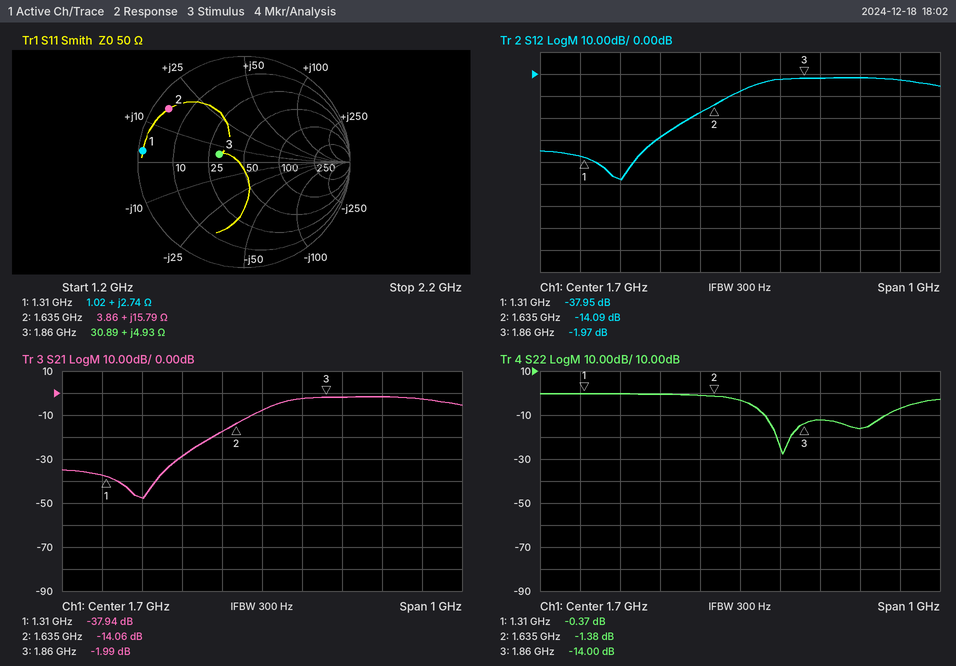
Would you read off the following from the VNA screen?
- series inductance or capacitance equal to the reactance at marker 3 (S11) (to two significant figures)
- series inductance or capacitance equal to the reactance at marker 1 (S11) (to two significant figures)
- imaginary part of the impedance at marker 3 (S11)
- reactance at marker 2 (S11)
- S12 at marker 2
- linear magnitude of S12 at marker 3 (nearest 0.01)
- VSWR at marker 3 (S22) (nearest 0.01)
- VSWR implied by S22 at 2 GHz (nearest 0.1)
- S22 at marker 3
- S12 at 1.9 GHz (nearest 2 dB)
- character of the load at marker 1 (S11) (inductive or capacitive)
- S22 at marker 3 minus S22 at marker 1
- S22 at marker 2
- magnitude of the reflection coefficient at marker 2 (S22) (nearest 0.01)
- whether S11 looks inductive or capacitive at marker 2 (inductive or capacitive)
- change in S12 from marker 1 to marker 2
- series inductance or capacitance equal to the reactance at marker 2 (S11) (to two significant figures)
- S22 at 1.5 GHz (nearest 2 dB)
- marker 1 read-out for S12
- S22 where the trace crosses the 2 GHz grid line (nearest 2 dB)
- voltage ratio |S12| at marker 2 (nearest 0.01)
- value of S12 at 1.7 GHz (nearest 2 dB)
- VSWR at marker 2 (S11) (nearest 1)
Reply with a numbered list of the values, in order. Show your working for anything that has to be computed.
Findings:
1. L = 4.93 Ω/(2π × 1.86 GHz) ≈ 422 pH, so 420 pH to two significant figures
2. L = 2.74 Ω/(2π × 1.31 GHz) ≈ 333 pH, so 330 pH to two significant figures
3. +4.93 Ω
4. +15.79 Ω
5. -14.09 dB
6. 10^(-1.97/20) ≈ 0.80
7. (1 + 0.1995)/(1 − 0.1995) ≈ 1.50
8. |Γ| = 10^(-16/20) = 0.1585; VSWR = (1 + 0.1585)/(1 − 0.1585) ≈ 1.4
9. -14.00 dB
10. -2 dB
11. inductive
12. -14 − (-0.37) = -13.63 dB
13. -1.38 dB
14. 10^(-1.38/20) ≈ 0.85
15. inductive
16. -14.09 − (-37.95) = 23.86 dB
17. L = 15.79 Ω/(2π × 1.635 GHz) ≈ 1.5 nH
18. 0 dB
19. -37.95 dB
20. -16 dB
21. 10^(-14.09/20) ≈ 0.20
22. -8 dB
23. 14
